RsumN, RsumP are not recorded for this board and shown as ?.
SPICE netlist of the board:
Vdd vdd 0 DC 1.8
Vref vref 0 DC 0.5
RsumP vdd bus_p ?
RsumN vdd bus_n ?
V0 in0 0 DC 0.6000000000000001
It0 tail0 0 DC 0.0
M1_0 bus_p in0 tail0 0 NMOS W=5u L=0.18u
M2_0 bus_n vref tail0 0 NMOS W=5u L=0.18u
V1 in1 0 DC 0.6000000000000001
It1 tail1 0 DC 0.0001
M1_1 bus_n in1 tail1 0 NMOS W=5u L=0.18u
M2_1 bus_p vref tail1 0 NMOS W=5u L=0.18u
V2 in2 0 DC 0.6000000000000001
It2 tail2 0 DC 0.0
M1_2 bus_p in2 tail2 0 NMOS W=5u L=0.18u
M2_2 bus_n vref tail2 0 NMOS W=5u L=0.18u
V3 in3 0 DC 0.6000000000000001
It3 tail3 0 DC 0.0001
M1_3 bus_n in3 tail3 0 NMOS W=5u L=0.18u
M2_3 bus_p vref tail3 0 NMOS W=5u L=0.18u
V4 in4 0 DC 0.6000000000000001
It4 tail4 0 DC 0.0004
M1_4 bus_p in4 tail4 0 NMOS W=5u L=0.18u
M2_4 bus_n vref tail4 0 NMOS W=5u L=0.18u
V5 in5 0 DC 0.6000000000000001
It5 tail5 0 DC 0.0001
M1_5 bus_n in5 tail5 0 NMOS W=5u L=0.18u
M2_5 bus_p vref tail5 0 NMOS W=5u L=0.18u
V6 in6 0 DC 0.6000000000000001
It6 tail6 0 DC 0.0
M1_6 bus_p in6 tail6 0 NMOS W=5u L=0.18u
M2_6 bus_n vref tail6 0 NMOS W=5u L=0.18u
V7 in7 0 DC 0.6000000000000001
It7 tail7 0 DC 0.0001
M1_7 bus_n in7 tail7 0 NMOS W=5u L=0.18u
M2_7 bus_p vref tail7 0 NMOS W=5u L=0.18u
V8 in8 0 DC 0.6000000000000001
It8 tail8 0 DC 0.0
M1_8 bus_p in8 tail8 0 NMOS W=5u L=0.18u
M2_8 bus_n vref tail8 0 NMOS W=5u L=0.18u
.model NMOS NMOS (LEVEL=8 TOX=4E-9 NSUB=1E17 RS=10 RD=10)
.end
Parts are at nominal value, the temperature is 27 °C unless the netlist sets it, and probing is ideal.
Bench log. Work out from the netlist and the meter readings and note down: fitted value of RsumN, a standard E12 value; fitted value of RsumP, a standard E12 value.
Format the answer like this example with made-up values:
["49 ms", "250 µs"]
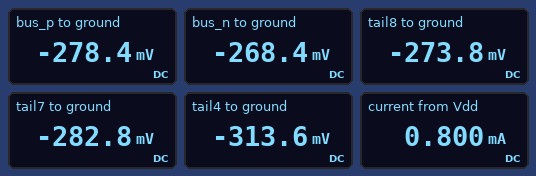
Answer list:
["3.3 kΩ", "12 kΩ"]
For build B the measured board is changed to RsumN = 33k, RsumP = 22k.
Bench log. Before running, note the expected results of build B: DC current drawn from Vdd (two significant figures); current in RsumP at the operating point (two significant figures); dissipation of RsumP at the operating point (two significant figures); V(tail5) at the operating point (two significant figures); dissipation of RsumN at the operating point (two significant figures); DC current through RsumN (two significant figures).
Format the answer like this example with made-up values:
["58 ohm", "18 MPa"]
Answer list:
["180 µA", "110 µA", "250 µW", "-550 mV", "170 µW", "71 µA"]
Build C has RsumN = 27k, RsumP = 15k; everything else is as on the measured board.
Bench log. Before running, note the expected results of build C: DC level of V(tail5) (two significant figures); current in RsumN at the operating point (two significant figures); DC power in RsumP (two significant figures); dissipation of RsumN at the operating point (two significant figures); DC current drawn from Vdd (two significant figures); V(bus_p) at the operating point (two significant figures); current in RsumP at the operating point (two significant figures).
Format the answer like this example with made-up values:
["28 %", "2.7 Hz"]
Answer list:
["-550 mV", "87 µA", "370 µW", "200 µW", "240 µA", "-540 mV", "160 µA"]
